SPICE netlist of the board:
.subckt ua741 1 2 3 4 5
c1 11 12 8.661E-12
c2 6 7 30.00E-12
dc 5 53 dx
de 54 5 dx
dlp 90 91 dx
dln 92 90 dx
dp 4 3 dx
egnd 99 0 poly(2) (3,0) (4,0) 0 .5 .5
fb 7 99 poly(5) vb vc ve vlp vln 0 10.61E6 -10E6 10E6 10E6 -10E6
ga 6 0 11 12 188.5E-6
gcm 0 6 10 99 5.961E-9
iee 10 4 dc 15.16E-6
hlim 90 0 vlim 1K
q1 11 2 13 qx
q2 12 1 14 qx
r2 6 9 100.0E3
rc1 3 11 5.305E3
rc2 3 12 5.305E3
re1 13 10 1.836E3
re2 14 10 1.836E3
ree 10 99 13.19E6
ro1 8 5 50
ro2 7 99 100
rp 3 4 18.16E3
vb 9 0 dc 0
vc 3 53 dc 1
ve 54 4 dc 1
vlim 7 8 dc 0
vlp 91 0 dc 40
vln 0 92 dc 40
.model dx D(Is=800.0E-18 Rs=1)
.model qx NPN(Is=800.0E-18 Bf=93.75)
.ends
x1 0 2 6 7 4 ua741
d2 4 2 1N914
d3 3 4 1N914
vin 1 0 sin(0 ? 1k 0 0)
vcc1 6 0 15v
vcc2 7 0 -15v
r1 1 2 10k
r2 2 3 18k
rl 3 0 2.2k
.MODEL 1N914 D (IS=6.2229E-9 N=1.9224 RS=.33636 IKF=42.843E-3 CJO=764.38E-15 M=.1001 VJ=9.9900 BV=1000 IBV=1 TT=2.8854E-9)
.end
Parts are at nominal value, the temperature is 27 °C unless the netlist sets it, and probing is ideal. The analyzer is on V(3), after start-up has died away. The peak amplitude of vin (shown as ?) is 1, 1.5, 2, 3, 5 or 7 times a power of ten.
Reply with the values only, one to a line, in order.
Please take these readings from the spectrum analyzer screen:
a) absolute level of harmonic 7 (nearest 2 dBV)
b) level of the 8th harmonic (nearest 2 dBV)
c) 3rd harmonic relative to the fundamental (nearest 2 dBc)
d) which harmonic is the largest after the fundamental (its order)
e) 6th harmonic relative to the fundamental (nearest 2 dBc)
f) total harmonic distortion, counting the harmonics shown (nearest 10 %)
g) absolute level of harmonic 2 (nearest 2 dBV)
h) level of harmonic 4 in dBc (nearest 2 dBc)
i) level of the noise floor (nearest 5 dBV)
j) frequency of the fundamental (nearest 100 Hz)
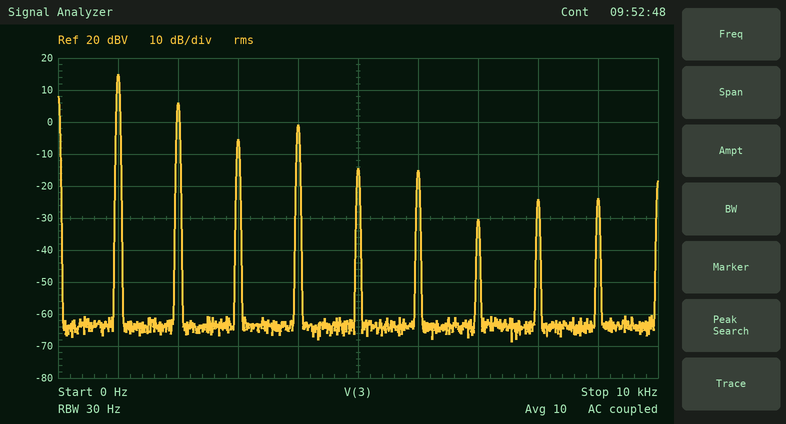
-30 dBV
-24 dBV
-20 dBc
2
-30 dBc
40 %
6 dBV
-16 dBc
-65 dBV
1.0 kHz
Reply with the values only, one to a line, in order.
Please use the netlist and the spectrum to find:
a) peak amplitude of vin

10 V
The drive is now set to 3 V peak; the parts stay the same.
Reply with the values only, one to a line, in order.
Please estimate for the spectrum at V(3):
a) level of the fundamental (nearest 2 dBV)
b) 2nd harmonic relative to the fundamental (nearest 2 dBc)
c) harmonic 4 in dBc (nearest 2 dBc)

6 dBV
-8 dBc
-22 dBc
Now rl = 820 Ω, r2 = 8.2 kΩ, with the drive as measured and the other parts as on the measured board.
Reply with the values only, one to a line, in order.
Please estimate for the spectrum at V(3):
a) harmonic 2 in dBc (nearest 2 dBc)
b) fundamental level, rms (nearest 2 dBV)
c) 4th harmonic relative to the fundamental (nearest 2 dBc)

-8 dBc
10 dBV
-22 dBc
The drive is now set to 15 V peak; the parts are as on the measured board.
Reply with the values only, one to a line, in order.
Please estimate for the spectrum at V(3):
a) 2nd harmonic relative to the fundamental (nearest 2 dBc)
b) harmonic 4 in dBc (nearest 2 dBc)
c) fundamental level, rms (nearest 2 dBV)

-12 dBc
-14 dBc
16 dBV
